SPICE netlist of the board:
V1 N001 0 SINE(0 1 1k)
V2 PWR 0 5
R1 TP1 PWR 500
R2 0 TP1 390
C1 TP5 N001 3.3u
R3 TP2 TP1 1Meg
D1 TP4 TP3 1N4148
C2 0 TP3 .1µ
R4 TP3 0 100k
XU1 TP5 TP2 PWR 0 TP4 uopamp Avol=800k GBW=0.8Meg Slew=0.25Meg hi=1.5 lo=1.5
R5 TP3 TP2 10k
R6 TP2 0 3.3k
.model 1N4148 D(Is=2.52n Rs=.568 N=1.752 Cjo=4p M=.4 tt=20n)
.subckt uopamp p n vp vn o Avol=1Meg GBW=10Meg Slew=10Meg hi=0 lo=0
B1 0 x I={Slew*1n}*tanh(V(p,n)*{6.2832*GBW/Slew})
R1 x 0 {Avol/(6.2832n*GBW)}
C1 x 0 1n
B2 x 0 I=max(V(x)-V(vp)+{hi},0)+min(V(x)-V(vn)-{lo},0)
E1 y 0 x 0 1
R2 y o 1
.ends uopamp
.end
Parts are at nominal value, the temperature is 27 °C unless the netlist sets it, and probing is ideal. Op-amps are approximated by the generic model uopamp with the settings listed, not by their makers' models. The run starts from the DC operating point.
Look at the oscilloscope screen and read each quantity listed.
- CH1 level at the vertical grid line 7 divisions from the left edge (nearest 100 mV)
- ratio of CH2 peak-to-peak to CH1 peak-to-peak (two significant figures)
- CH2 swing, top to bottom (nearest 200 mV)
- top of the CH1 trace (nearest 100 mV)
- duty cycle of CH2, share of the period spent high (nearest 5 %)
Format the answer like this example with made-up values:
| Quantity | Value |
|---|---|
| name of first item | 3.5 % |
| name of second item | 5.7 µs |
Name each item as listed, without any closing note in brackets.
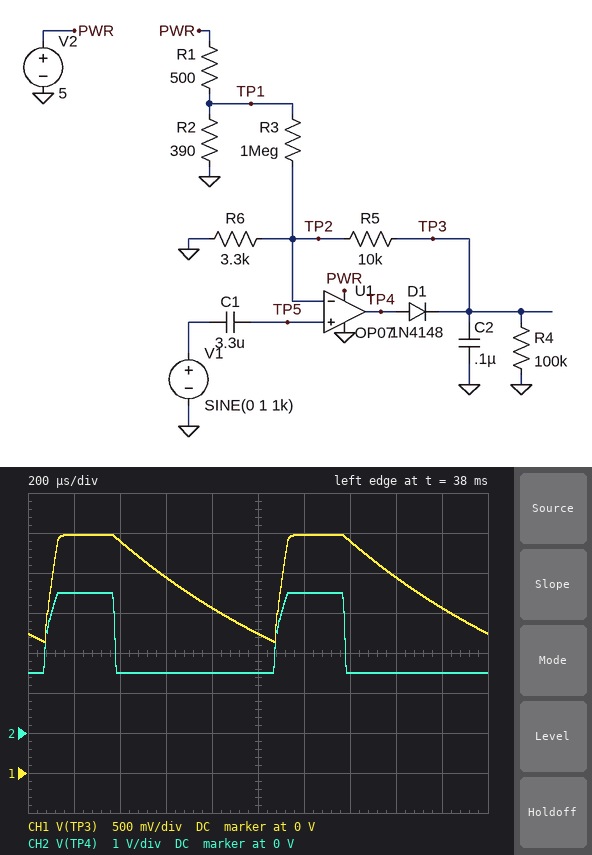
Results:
| Quantity | Value |
|---|---|
| CH1 level at the vertical grid line 7 divisions from the left edge | 2.9 V |
| ratio of CH2 peak-to-peak to CH1 peak-to-peak | 1.5 |
| CH2 swing, top to bottom | 2.0 V |
| top of the CH1 trace | 3.0 V |
| duty cycle of CH2, share of the period spent high | 30 % |
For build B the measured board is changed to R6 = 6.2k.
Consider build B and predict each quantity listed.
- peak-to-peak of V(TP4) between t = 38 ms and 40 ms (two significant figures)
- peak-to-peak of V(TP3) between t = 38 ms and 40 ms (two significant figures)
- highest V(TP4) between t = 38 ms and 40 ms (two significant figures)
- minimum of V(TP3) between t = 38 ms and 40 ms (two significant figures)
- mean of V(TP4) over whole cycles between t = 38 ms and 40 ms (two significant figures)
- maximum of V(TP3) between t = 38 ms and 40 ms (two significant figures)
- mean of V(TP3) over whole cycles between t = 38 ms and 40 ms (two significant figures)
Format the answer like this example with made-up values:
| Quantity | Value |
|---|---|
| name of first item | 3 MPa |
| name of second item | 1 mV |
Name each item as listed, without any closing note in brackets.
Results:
| Quantity | Value |
|---|---|
| peak-to-peak of V(TP4) between t = 38 ms and 40 ms | 1.6 V |
| peak-to-peak of V(TP3) between t = 38 ms and 40 ms | 1.2 V |
| highest V(TP4) between t = 38 ms and 40 ms | 3.1 V |
| minimum of V(TP3) between t = 38 ms and 40 ms | 1.4 V |
| mean of V(TP4) over whole cycles between t = 38 ms and 40 ms | 1.8 V |
| maximum of V(TP3) between t = 38 ms and 40 ms | 2.6 V |
| mean of V(TP3) over whole cycles between t = 38 ms and 40 ms | 2.0 V |
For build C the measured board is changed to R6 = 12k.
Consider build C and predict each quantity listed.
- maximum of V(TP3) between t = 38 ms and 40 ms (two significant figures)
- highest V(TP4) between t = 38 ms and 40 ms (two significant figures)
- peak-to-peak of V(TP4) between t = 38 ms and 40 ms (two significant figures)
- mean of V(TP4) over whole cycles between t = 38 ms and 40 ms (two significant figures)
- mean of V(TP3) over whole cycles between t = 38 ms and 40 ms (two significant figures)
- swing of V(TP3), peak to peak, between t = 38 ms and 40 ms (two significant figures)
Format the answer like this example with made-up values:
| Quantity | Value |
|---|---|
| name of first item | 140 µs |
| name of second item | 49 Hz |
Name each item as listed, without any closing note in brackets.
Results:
| Quantity | Value |
|---|---|
| maximum of V(TP3) between t = 38 ms and 40 ms | 1.8 V |
| highest V(TP4) between t = 38 ms and 40 ms | 2.3 V |
| peak-to-peak of V(TP4) between t = 38 ms and 40 ms | 830 mV |
| mean of V(TP4) over whole cycles between t = 38 ms and 40 ms | 1.6 V |
| mean of V(TP3) over whole cycles between t = 38 ms and 40 ms | 1.5 V |
| swing of V(TP3), peak to peak, between t = 38 ms and 40 ms | 680 mV |
